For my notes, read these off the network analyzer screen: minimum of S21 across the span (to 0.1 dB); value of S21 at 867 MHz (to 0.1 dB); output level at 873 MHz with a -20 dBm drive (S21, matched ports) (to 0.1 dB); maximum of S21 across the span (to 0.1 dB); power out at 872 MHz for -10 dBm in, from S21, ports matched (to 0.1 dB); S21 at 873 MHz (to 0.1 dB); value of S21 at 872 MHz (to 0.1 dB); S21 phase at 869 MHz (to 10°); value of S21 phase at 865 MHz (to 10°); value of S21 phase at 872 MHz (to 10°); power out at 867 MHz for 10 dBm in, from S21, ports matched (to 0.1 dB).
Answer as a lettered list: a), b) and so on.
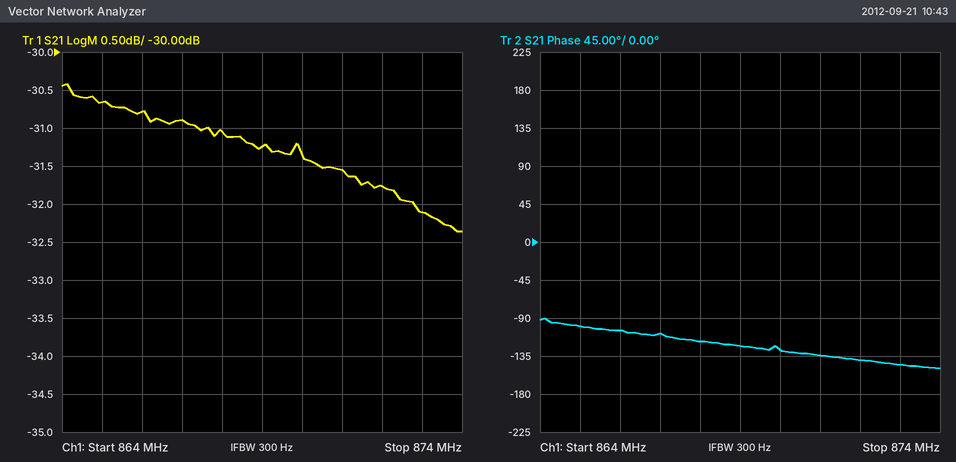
a) -32.4 dB
b) -30.9 dB
c) -52.1 dBm
d) -30.4 dB
e) -41.8 dBm
f) -32.1 dB
g) -31.8 dB
h) -120°
i) -100°
j) -140°
k) -20.9 dBm
